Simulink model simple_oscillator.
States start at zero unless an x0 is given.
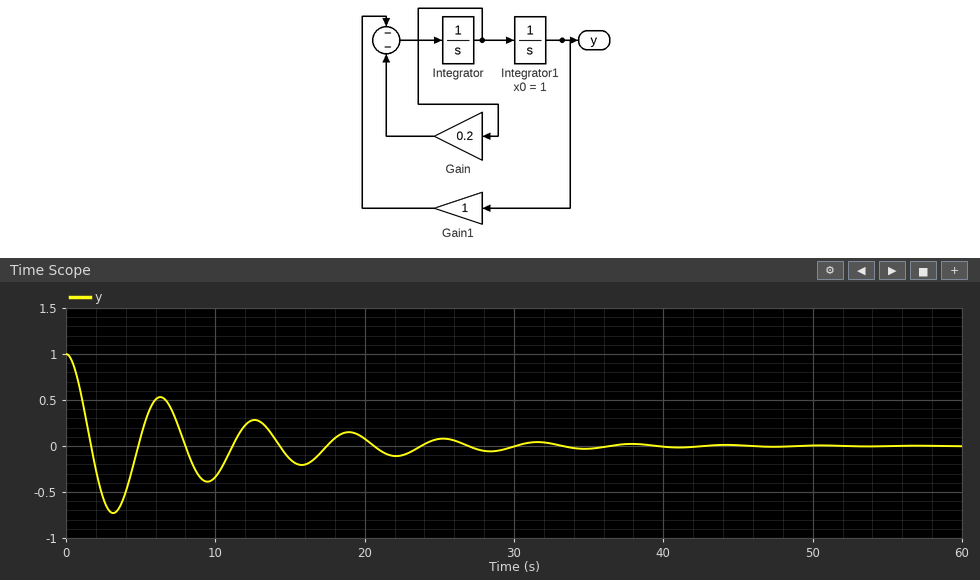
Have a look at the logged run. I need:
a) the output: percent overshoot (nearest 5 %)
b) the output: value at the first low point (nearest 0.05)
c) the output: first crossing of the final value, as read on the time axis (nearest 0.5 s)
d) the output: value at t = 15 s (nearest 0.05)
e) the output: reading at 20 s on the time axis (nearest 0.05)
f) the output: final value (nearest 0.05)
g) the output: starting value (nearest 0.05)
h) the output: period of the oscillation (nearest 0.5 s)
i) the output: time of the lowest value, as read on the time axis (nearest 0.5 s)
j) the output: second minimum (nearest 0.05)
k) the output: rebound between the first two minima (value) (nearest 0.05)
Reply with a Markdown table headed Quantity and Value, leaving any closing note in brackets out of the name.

| Quantity | Value |
|---|---|
| the output: percent overshoot | 75 % |
| the output: value at the first low point | -0.75 |
| the output: first crossing of the final value, as read on the time axis | 1.5 s |
| the output: value at t = 15 s | -0.15 |
| the output: reading at 20 s on the time axis | 0.10 |
| the output: final value | 0.00 |
| the output: starting value | 1.00 |
| the output: period of the oscillation | 6.5 s |
| the output: time of the lowest value, as read on the time axis | 3.0 s |
| the output: second minimum | -0.40 |
| the output: rebound between the first two minima (value) | 0.55 |
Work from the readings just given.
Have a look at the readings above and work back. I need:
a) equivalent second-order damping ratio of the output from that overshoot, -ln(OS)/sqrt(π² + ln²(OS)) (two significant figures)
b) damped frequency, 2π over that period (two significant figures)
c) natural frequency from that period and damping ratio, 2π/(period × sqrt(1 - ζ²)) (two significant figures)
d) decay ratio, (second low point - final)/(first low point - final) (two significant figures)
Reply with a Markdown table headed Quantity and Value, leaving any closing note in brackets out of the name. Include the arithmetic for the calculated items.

| Quantity | Value |
|---|---|
| equivalent second-order damping ratio of the output from that overshoot, -ln(OS)/sqrt(π² + ln²(OS)) | ln(0.75) = -0.288; 0.288 / sqrt(9.870 + 0.083) = 0.091 |
| damped frequency, 2π over that period | 2π / 6.5 = 0.97 rad/s |
| natural frequency from that period and damping ratio, 2π/(period × sqrt(1 - ζ²)) | 2π / (6.5 × sqrt(1 - 0.091²)) = 0.97 rad/s |
| decay ratio, (second low point - final)/(first low point - final) | (-0.4 - 0) / (-0.75 - 0) = 0.53 |
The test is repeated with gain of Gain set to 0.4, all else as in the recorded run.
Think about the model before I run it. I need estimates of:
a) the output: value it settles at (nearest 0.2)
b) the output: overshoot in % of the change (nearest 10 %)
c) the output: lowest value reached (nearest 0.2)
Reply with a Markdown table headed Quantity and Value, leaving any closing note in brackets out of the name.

| Quantity | Value |
|---|---|
| the output: value it settles at | 0.0 |
| the output: overshoot in % of the change | 50 % |
| the output: lowest value reached | -0.6 |
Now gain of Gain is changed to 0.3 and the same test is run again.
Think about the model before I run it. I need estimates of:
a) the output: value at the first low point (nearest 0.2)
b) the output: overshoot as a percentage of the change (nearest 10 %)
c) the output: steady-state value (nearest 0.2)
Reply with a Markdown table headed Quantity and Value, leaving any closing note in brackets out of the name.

| Quantity | Value |
|---|---|
| the output: value at the first low point | -0.6 |
| the output: overshoot as a percentage of the change | 60 % |
| the output: steady-state value | 0.0 |
